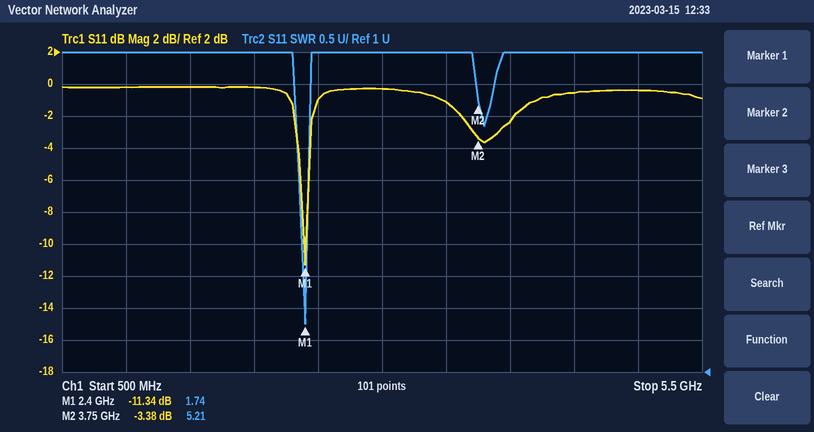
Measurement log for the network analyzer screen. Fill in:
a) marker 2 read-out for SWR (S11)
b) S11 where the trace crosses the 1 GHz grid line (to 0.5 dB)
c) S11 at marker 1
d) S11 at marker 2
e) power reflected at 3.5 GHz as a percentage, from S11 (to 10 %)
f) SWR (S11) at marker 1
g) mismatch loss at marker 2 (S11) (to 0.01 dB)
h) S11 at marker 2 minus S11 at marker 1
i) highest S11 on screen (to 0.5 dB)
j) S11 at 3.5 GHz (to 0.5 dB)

5.21
0.0 dB
-11.34 dB
-3.38 dB
80 %
1.74
2.67 dB
7.96 dB
0.0 dB
-1.0 dB
